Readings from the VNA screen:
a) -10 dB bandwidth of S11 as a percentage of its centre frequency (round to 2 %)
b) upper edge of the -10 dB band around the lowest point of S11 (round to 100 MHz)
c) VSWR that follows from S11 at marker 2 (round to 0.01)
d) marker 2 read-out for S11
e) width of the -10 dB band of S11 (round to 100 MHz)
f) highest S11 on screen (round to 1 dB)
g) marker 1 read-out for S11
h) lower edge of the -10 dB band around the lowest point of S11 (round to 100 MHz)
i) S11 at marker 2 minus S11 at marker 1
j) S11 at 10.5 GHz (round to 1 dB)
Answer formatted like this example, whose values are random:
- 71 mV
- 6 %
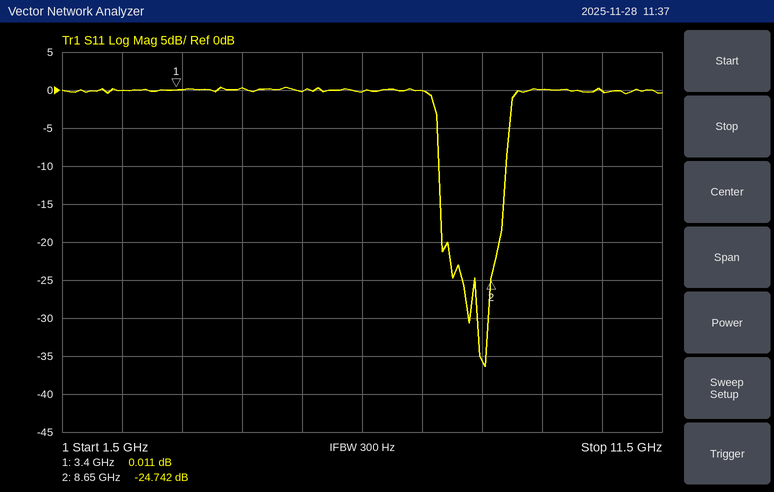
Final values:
- 14 %
- 8.9 GHz
- 1.12
- -24.742 dB
- 1.1 GHz
- 0 dB
- 0.011 dB
- 7.8 GHz
- -24.753 dB
- 0 dB
